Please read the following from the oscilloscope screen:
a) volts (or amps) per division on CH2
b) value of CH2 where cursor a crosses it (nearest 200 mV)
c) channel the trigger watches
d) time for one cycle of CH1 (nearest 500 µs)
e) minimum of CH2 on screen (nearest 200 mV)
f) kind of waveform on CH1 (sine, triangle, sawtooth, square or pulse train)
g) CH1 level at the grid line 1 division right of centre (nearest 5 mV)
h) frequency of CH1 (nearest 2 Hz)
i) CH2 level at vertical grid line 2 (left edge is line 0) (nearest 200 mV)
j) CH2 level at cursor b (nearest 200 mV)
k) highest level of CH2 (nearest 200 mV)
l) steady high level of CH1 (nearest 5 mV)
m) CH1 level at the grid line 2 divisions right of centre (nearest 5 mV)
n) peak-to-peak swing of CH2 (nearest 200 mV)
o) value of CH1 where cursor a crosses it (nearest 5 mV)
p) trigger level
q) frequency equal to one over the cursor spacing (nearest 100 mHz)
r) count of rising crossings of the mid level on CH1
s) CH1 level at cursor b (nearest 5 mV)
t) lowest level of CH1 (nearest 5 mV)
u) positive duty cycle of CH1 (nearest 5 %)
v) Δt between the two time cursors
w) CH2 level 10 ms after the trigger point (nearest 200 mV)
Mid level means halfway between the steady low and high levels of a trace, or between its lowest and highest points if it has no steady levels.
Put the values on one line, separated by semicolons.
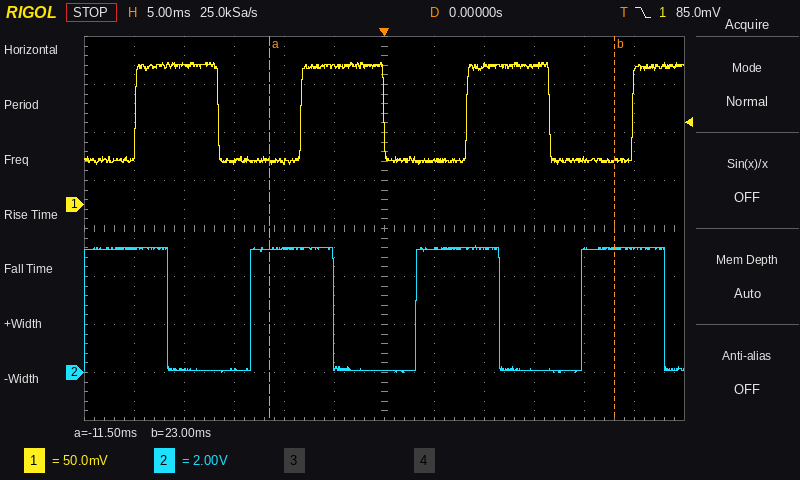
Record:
2 V; 5.2 V; CH1; 16.5 ms; 0.0 V; square; 45 mV; 60 Hz; 200 mV; 5.2 V; 5.2 V; 145 mV; 145 mV; 5.2 V; 45 mV; 85.0 mV; 29.0 Hz; 4; 45 mV; 40 mV; 50 %; 34.5 ms; 5.2 V
